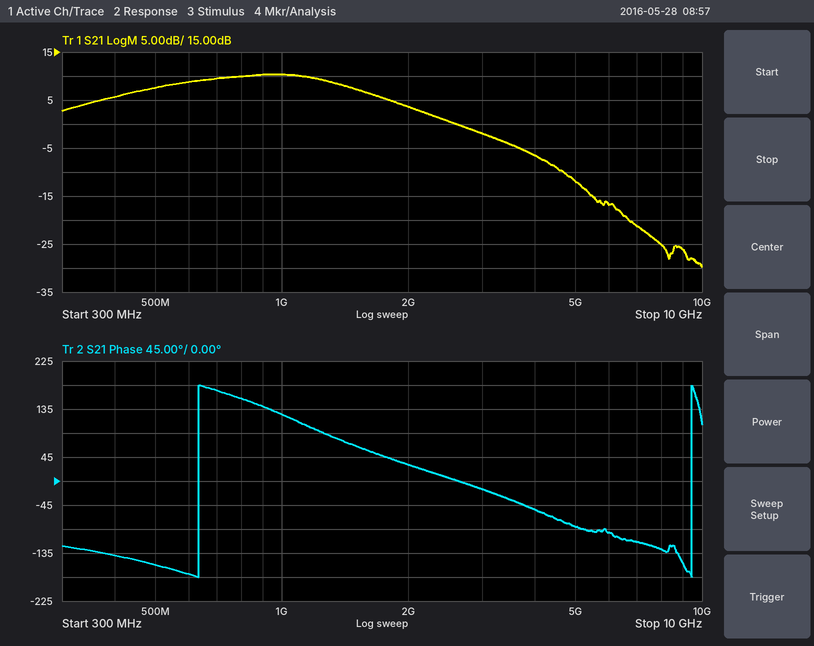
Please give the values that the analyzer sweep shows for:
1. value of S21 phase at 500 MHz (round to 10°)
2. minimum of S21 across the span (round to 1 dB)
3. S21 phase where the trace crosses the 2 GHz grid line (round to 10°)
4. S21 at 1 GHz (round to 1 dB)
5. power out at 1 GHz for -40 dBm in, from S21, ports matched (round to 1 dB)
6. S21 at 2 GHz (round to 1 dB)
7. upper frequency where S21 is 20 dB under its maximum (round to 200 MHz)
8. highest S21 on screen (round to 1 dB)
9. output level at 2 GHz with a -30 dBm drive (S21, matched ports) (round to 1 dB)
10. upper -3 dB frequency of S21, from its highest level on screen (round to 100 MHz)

-160°
-30 dB
30°
10 dB
-30 dBm
4 dB
4.6 GHz
10 dB
-26 dBm
1.5 GHz
